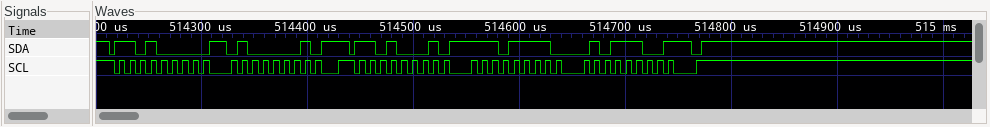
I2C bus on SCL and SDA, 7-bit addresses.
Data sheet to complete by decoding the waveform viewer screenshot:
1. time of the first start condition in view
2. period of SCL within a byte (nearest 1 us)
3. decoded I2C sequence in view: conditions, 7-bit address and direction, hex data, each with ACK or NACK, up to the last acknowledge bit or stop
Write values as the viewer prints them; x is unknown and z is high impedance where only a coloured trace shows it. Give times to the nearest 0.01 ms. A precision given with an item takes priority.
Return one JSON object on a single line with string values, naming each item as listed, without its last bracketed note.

{"time of the first start condition in view": "514.21 ms", "period of SCL within a byte": "10 us", "decoded I2C sequence in view: conditions, 7-bit address and direction, hex data, each with ACK or NACK, up to the last acknowledge bit or stop": "start, address 68 write ACK, 41 ACK, repeated start, address 68 read ACK, EF ACK, 5C NACK, stop"}
